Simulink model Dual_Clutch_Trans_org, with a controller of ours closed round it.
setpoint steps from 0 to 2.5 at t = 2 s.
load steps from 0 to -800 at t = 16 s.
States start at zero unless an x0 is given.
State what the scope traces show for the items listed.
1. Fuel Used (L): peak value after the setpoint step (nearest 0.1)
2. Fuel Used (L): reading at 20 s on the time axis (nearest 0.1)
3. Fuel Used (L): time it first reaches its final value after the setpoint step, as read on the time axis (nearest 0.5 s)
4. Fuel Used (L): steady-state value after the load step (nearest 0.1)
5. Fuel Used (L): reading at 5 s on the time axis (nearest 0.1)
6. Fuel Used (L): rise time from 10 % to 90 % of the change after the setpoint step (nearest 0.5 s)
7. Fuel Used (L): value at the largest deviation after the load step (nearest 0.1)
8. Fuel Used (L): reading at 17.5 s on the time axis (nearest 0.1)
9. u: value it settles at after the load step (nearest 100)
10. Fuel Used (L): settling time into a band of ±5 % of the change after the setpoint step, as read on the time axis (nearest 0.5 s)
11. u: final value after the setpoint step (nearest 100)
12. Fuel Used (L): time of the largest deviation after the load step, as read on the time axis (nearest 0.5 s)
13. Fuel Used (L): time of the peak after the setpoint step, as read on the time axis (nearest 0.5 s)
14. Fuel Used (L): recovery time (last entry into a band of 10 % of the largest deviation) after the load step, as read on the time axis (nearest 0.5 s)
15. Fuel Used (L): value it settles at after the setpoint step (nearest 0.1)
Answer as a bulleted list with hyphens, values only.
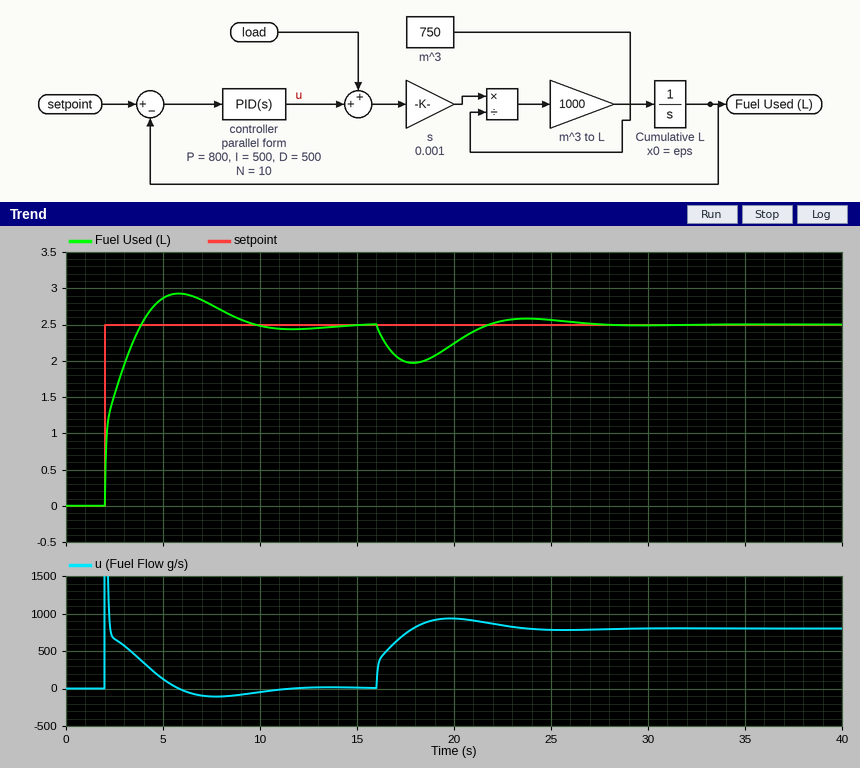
- 2.9
- 2.2
- 4.0 s
- 2.5
- 2.9
- 1.5 s
- 2.0
- 2.0
- 800
- 8.5 s
- 0
- 18.0 s
- 6.0 s
- 25.5 s
- 2.5
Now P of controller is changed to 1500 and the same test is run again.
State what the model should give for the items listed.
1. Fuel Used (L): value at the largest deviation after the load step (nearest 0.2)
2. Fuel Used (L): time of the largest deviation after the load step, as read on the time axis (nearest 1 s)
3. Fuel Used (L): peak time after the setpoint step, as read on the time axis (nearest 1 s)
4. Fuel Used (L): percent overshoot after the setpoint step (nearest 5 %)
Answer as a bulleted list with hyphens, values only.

- 2.2
- 18 s
- 5 s
- 10 %
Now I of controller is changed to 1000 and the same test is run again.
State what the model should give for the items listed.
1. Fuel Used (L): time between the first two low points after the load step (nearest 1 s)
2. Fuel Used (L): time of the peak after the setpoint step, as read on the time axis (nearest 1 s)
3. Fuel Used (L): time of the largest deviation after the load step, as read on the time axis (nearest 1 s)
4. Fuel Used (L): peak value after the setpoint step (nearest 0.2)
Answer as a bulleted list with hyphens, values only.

- 8 s
- 5 s
- 17 s
- 3.0
